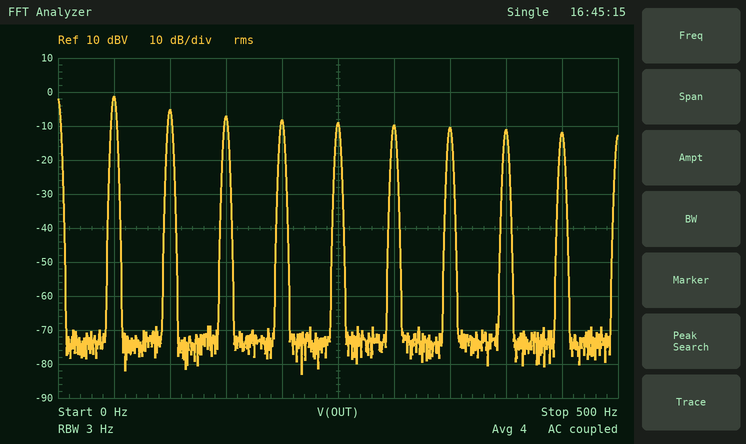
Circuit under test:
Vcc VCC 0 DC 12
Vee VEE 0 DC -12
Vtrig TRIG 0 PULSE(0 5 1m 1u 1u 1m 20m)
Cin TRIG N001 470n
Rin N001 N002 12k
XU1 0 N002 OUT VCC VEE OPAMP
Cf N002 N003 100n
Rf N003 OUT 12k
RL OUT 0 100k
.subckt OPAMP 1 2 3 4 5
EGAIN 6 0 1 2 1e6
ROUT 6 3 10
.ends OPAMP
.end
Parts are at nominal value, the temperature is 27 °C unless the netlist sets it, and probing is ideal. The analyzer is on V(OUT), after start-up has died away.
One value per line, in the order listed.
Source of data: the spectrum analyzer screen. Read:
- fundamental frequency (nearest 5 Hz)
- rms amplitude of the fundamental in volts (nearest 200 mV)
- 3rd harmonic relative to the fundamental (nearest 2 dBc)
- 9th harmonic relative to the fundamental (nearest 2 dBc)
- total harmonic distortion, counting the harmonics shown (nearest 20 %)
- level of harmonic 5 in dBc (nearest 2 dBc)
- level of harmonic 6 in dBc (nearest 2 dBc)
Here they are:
50 Hz
800 mV
-6 dBc
-10 dBc
120 %
-8 dBc
-8 dBc
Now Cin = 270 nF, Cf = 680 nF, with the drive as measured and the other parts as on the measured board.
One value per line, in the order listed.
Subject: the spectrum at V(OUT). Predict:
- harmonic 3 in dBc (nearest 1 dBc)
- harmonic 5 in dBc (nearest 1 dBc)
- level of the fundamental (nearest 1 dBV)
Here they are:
2 dBc
1 dBc
-11 dBV
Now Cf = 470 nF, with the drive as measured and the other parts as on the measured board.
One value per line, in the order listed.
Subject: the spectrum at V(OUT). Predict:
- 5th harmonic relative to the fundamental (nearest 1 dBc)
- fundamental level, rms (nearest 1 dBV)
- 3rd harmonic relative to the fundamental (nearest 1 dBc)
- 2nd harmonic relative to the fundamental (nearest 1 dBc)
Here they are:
-1 dBc
-9 dBV
0 dBc
0 dBc
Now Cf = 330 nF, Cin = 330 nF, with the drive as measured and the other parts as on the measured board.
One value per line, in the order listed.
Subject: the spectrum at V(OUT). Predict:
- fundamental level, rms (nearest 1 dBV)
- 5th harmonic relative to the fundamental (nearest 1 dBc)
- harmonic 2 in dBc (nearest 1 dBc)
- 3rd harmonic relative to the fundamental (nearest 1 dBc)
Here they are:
-9 dBV
-1 dBc
0 dBc
0 dBc
